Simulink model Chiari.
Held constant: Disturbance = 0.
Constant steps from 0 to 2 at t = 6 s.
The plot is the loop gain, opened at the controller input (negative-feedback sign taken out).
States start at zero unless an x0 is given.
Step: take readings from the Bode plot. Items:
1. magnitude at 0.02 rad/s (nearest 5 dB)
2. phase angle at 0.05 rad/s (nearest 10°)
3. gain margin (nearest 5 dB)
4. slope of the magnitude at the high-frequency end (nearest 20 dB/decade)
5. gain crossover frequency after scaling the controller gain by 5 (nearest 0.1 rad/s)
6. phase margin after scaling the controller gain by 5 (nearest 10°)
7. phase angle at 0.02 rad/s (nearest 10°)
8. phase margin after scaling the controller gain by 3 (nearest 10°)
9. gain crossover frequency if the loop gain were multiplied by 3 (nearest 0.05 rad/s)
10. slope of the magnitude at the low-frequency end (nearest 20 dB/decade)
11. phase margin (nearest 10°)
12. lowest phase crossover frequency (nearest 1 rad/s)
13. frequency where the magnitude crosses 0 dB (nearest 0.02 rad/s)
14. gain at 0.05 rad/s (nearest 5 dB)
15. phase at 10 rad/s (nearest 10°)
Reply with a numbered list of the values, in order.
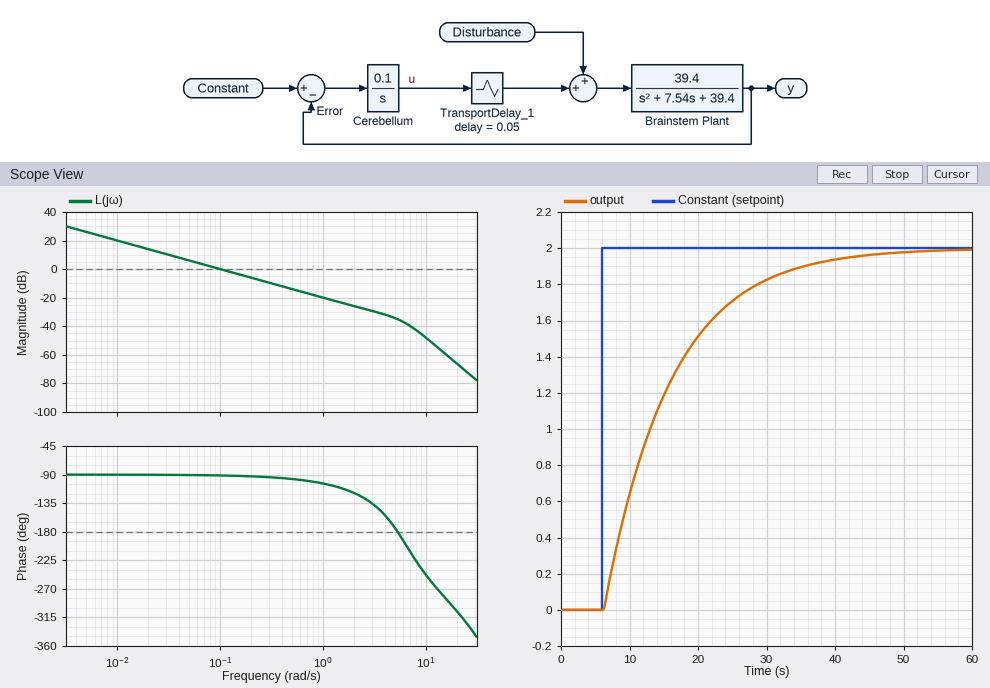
1. 15 dB
2. -90°
3. 35 dB
4. -60 dB/decade
5. 0.5 rad/s
6. 80°
7. -90°
8. 90°
9. 0.30 rad/s
10. -20 dB/decade
11. 90°
12. 5 rad/s
13. 0.10 rad/s
14. 5 dB
15. -250°
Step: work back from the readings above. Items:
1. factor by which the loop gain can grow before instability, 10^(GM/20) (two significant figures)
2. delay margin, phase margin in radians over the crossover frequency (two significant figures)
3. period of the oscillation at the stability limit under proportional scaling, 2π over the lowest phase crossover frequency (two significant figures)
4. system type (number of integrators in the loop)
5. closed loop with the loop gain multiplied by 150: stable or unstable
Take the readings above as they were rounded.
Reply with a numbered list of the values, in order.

1. 56
2. 16 s
3. 1.3 s
4. 1
5. unstable
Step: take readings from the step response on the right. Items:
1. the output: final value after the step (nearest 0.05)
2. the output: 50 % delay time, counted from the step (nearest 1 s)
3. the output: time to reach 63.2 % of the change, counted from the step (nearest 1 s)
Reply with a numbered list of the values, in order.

1. 2.00
2. 7 s
3. 10 s
